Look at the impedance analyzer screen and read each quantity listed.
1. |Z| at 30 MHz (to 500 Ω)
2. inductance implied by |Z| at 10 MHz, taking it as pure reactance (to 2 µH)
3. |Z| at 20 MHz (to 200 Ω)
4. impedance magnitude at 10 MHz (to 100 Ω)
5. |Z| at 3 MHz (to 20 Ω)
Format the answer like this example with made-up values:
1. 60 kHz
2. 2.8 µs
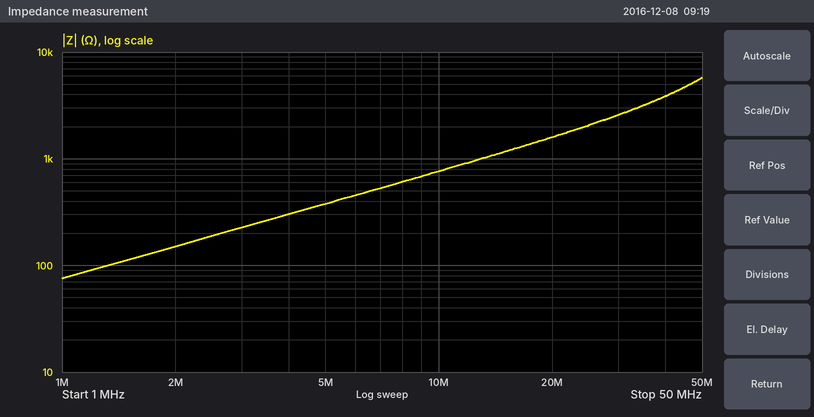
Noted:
1. 2.5 kΩ
2. 12 µH
3. 1.6 kΩ
4. 800 Ω
5. 220 Ω
